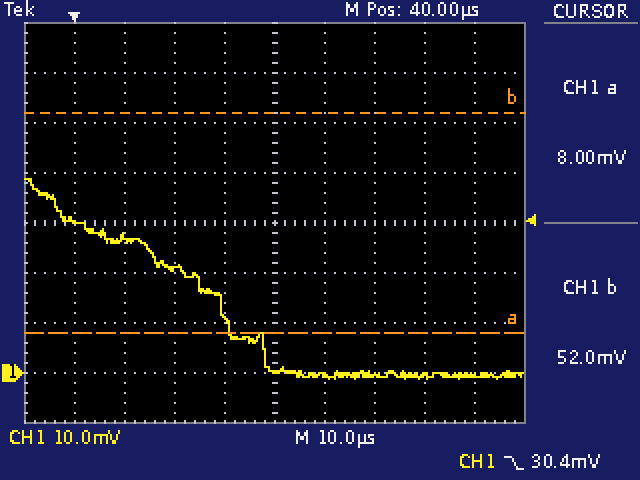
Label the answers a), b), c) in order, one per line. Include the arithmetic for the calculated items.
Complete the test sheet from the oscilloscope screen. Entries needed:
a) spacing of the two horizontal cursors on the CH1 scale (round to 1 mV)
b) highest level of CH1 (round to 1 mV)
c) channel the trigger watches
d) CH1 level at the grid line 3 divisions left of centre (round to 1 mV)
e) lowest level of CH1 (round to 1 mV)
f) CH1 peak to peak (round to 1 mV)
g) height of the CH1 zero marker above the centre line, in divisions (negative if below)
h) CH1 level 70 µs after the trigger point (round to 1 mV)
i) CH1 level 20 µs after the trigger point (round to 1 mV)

a) 44 mV
b) 39 mV
c) CH1
d) 27 mV
e) -1 mV
f) 39 mV − (-1 mV) = 40 mV
g) -3.0 div
h) -1 mV
i) 21 mV
